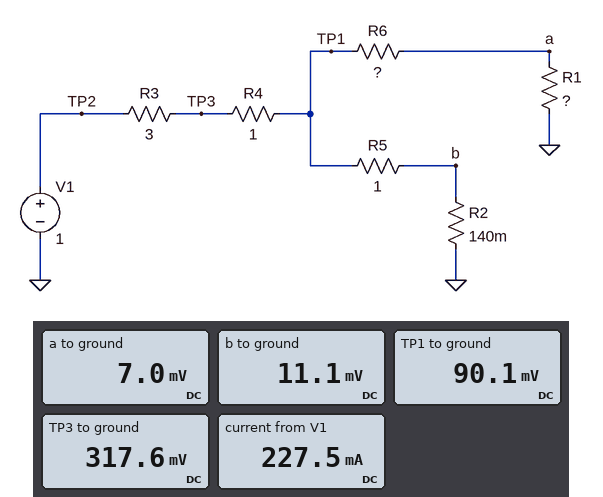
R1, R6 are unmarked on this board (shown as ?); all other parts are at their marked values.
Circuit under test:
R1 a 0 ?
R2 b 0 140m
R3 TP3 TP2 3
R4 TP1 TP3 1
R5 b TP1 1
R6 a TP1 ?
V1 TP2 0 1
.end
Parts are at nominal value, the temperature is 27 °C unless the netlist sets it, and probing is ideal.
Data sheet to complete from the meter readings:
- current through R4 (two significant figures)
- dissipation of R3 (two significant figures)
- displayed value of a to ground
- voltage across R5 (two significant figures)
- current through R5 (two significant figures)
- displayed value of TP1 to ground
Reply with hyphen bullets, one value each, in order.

- 230 mA
- 160 mW
- 7.0 mV
- 79 mV
- 79 mA
- 90.1 mV
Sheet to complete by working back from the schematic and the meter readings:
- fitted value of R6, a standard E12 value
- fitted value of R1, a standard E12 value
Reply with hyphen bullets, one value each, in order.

- 0.56 Ω
- 0.047 Ω
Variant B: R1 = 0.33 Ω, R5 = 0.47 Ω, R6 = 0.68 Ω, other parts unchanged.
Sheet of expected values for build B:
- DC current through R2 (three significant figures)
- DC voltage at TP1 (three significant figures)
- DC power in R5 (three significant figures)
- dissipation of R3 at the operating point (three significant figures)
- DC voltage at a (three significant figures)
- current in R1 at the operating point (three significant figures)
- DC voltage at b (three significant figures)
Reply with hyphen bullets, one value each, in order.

- 142 mA
- 86.8 mV
- 9.52 mW
- 156 mW
- 28.4 mV
- 86.0 mA
- 19.9 mV
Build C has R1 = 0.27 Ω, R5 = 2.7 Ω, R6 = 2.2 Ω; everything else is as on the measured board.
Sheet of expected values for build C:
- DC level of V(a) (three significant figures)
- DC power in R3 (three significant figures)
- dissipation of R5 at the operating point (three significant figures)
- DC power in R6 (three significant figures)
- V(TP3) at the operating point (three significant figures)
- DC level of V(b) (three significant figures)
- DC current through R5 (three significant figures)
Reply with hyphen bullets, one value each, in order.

- 27.1 mV
- 106 mW
- 20.6 mW
- 22.2 mW
- 436 mV
- 12.2 mV
- 87.4 mA
